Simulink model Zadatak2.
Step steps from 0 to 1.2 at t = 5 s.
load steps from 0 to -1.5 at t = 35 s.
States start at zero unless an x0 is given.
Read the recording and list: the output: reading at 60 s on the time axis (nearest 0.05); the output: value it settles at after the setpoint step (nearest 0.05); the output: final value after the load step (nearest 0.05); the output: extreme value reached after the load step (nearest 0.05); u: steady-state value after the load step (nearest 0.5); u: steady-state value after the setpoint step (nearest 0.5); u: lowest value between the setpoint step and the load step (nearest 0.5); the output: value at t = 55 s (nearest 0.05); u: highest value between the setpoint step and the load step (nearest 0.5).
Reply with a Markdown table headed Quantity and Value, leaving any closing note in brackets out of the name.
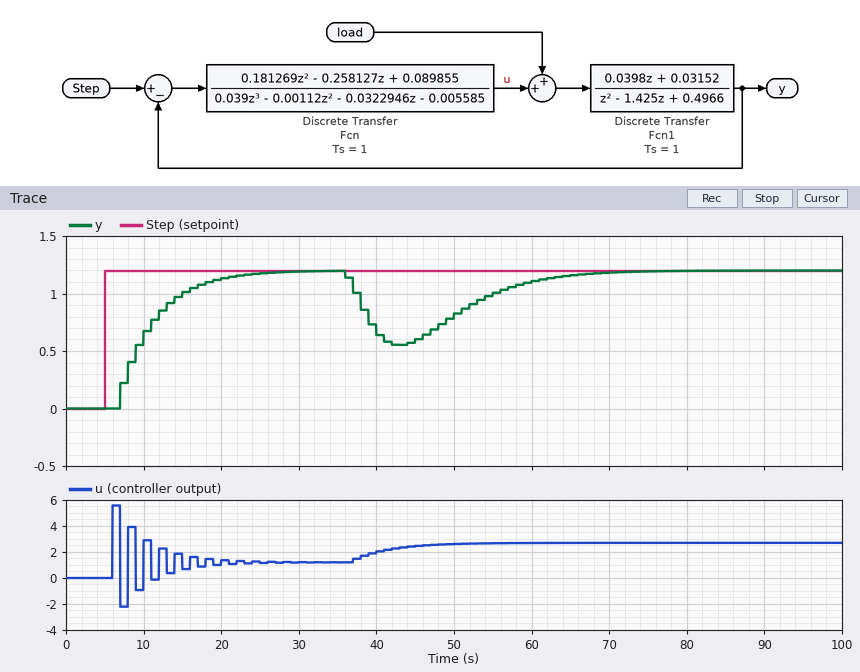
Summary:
| Quantity | Value |
|---|---|
| the output: reading at 60 s on the time axis | 1.10 |
| the output: value it settles at after the setpoint step | 1.20 |
| the output: final value after the load step | 1.20 |
| the output: extreme value reached after the load step | 0.55 |
| u: steady-state value after the load step | 2.5 |
| u: steady-state value after the setpoint step | 1.0 |
| u: lowest value between the setpoint step and the load step | -2.0 |
| the output: value at t = 55 s | 1.00 |
| u: highest value between the setpoint step and the load step | 5.5 |
